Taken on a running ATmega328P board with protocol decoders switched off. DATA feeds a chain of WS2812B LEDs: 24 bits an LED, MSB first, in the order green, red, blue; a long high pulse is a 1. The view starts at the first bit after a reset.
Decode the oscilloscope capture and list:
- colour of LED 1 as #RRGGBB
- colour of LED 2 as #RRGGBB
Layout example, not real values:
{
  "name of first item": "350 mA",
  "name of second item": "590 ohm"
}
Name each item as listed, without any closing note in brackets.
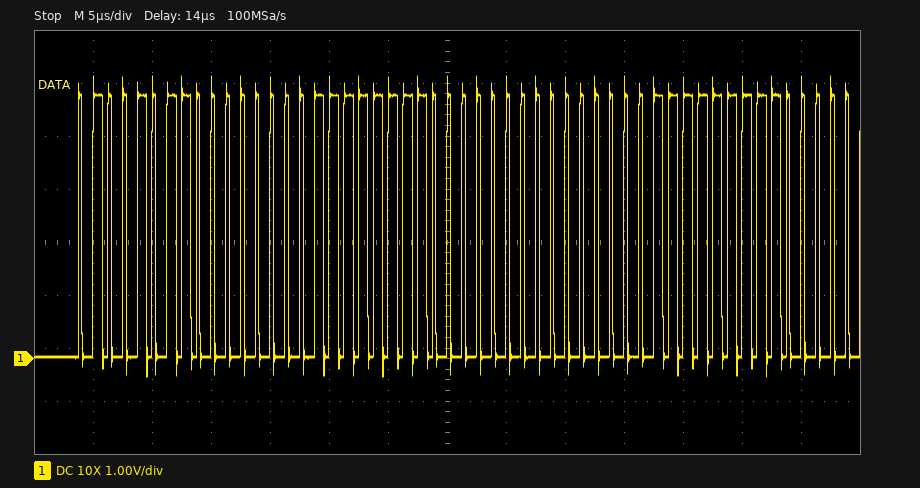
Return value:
{
  "colour of LED 1 as #RRGGBB": "#004BFF",
  "colour of LED 2 as #RRGGBB": "#0100FF"
}
